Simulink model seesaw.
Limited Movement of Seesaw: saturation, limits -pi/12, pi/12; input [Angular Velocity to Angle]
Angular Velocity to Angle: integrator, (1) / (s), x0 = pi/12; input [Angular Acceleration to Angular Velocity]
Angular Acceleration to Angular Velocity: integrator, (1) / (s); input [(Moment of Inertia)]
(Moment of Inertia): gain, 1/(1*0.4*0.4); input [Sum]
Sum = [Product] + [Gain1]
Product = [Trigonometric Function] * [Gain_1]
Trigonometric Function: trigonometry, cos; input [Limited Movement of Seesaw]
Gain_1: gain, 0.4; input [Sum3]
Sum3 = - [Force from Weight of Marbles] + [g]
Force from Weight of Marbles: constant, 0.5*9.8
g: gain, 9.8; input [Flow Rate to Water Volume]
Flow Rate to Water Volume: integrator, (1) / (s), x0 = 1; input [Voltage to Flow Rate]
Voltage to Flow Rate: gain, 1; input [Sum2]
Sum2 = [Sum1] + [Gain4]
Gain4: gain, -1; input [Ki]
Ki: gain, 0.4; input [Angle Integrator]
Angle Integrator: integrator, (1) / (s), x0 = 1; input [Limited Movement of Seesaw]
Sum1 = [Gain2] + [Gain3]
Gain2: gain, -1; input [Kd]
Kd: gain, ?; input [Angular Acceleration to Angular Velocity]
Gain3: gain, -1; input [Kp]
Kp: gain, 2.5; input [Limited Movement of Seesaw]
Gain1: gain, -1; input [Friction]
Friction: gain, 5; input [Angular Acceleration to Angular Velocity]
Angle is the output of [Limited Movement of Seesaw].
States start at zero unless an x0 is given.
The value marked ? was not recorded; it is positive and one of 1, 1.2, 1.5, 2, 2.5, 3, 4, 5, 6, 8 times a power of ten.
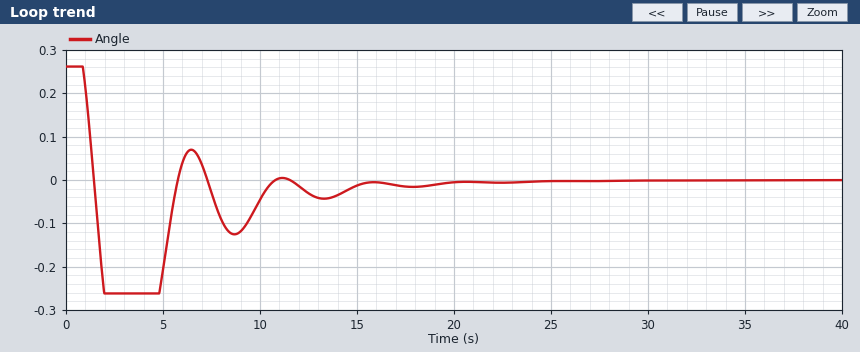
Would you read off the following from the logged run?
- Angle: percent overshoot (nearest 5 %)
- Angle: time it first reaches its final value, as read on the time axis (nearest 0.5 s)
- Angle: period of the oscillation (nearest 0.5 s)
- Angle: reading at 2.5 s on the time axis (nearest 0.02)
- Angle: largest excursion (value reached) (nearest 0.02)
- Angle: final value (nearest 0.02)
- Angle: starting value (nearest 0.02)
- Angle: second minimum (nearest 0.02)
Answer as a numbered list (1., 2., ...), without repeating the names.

1. 100 %
2. 1.5 s
3. 5.5 s
4. -0.26
5. -0.26
6. 0.00
7. 0.26
8. -0.12
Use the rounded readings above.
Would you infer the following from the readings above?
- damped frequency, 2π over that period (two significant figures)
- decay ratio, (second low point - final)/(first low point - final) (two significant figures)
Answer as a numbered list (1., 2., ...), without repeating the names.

1. 1.1 rad/s
2. 0.46
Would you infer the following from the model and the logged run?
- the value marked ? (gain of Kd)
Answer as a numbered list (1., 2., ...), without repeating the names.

1. 1
